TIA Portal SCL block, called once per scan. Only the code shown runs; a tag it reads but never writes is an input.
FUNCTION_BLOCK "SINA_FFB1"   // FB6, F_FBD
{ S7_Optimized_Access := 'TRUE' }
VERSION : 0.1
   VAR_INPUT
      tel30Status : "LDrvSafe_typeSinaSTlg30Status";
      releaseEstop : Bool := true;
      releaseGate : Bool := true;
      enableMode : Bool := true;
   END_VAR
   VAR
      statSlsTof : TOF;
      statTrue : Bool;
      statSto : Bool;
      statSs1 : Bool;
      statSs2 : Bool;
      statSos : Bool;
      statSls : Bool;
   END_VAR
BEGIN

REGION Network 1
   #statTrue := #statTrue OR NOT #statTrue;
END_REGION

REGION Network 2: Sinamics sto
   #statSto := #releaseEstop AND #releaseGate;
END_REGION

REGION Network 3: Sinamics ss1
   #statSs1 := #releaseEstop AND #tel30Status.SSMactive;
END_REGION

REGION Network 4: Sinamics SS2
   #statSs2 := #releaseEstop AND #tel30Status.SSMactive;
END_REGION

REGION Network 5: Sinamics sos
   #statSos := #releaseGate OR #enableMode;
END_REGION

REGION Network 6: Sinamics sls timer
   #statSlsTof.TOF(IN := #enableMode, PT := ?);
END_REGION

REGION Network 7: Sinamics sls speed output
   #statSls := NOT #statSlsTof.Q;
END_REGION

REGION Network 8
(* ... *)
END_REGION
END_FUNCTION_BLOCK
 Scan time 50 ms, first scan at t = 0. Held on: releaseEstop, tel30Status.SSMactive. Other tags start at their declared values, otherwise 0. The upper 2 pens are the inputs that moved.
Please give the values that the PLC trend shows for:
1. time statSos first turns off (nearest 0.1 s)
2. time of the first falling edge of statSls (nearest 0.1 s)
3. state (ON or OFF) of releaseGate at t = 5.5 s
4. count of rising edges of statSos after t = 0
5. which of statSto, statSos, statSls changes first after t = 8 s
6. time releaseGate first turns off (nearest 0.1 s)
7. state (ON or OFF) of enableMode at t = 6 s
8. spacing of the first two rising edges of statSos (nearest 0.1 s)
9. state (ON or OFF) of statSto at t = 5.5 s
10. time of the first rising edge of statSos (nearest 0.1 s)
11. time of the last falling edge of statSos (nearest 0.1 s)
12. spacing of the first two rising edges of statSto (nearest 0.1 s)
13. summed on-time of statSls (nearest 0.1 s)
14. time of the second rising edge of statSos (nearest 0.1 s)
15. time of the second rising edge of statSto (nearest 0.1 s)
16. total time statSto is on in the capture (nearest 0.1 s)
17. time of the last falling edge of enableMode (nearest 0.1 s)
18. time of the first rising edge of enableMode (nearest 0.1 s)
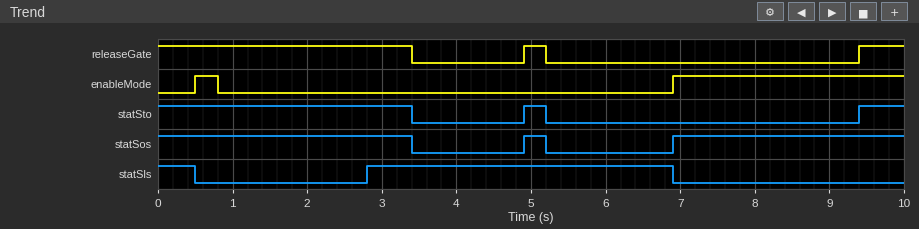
3.4 s
0.5 s
OFF
2
statSto
3.4 s
OFF
2.0 s
OFF
4.9 s
5.2 s
4.5 s
4.6 s
6.9 s
9.4 s
4.3 s
0.8 s
0.5 s
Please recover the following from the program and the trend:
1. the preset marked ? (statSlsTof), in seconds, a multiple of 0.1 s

2.0 s
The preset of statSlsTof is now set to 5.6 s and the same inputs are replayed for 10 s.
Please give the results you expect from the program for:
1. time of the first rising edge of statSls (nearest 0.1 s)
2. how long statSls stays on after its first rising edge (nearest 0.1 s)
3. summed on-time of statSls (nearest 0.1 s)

6.4 s
0.5 s
1.0 s
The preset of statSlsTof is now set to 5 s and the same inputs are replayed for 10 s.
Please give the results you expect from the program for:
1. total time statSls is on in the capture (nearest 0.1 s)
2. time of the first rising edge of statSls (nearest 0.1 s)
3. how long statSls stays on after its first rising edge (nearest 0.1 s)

1.6 s
5.8 s
1.1 s
